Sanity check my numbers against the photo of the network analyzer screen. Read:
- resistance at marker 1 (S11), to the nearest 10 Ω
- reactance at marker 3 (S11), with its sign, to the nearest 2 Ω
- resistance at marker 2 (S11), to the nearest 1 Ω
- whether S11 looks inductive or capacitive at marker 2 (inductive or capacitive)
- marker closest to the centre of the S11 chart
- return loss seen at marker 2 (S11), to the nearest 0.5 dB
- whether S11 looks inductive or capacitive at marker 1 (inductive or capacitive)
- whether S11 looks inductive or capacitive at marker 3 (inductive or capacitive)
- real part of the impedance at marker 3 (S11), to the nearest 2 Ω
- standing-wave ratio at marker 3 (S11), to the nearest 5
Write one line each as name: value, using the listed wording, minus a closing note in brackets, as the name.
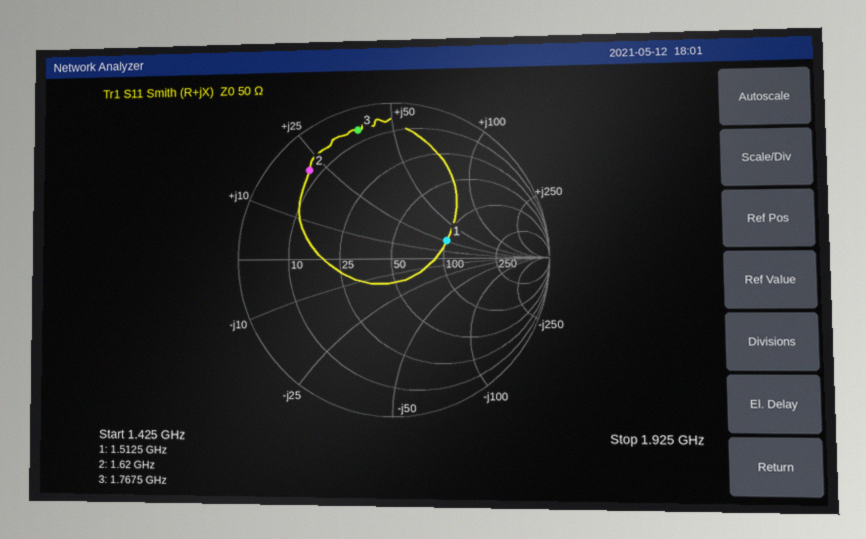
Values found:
resistance at marker 1 (S11), to the nearest 10 Ω: 100 Ω
reactance at marker 3 (S11), with its sign, to the nearest 2 Ω: +38 Ω
resistance at marker 2 (S11), to the nearest 1 Ω: 7 Ω
whether S11 looks inductive or capacitive at marker 2: inductive
marker closest to the centre of the S11 chart: marker 1
return loss seen at marker 2 (S11), to the nearest 0.5 dB: 2.0 dB
whether S11 looks inductive or capacitive at marker 1: inductive
whether S11 looks inductive or capacitive at marker 3: inductive
real part of the impedance at marker 3 (S11), to the nearest 2 Ω: 6 Ω
standing-wave ratio at marker 3 (S11), to the nearest 5: 15
